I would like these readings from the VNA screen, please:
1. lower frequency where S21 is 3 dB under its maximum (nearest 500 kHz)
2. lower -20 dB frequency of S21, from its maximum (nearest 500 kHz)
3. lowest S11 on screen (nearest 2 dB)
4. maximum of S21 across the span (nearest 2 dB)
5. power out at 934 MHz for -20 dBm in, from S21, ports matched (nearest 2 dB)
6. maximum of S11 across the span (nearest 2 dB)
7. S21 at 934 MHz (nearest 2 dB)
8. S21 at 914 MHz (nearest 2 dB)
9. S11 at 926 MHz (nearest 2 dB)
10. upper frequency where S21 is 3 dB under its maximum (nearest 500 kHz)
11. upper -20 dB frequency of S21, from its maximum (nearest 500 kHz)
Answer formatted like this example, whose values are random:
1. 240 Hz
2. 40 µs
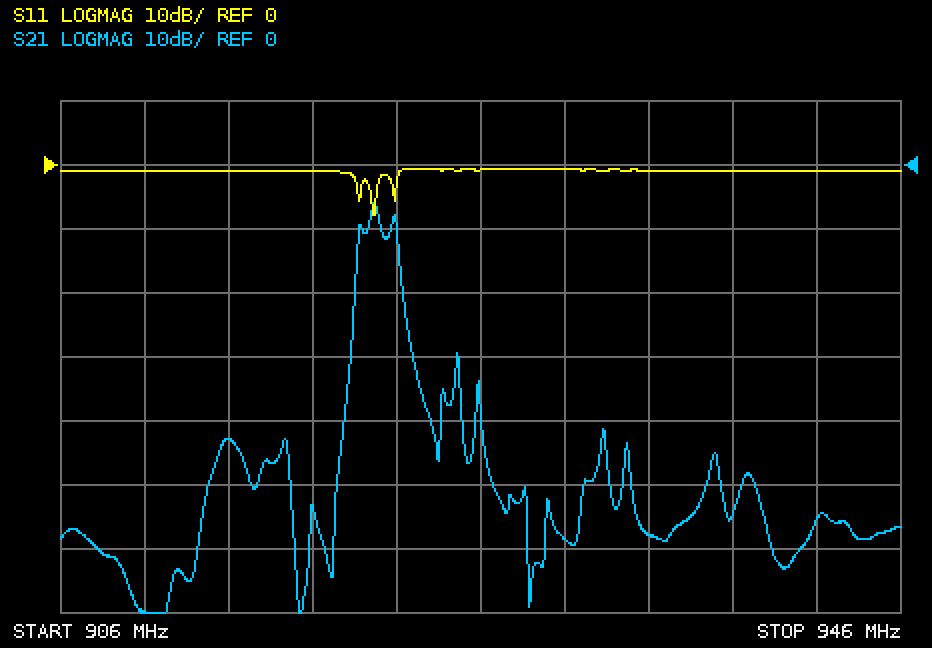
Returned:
1. 920.5 MHz
2. 920.0 MHz
3. -8 dB
4. -6 dB
5. -78 dBm
6. 0 dB
7. -58 dB
8. -42 dB
9. 0 dB
10. 921.0 MHz
11. 922.5 MHz
